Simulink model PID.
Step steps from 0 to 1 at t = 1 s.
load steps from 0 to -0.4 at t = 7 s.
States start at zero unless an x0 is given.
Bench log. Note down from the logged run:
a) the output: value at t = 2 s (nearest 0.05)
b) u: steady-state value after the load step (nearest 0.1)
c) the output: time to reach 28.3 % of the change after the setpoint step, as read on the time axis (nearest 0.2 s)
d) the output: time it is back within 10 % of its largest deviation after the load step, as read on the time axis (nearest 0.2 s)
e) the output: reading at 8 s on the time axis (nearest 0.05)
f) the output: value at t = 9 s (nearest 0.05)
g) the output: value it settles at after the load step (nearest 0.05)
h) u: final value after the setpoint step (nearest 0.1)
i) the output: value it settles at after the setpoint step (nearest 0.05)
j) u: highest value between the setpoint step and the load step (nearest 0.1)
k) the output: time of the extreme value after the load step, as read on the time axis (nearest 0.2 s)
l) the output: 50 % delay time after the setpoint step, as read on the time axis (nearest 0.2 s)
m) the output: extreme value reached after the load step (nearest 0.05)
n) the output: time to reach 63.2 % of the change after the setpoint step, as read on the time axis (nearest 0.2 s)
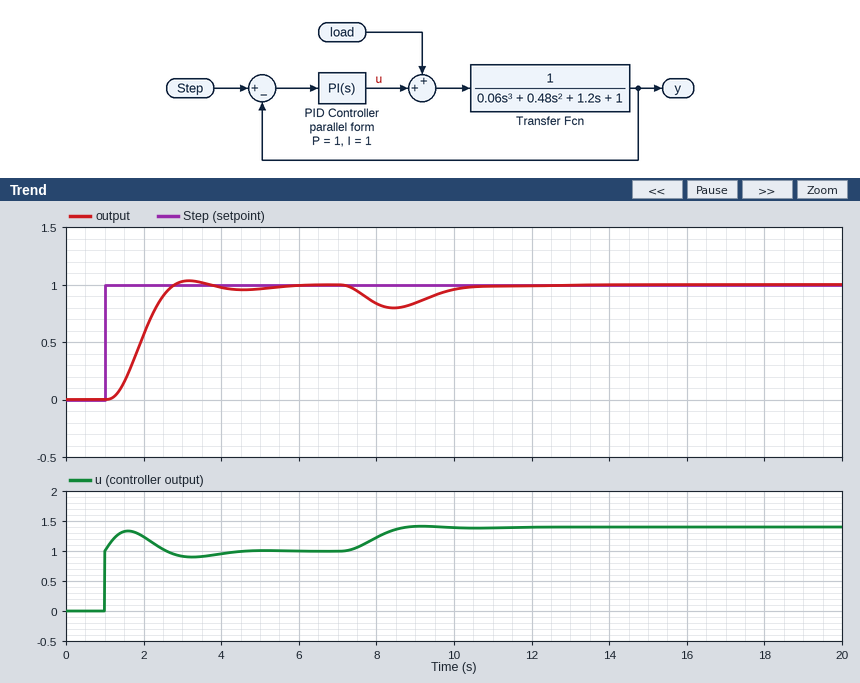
0.55
1.4
1.6 s
10.6 s
0.85
0.85
1.00
1.0
1.00
1.3
8.4 s
2.0 s
0.80
2.0 s
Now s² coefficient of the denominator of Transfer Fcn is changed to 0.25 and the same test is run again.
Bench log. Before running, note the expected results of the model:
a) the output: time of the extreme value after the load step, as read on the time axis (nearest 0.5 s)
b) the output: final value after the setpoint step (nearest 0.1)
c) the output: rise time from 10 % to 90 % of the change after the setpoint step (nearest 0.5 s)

8.0 s
1.0
2.0 s
